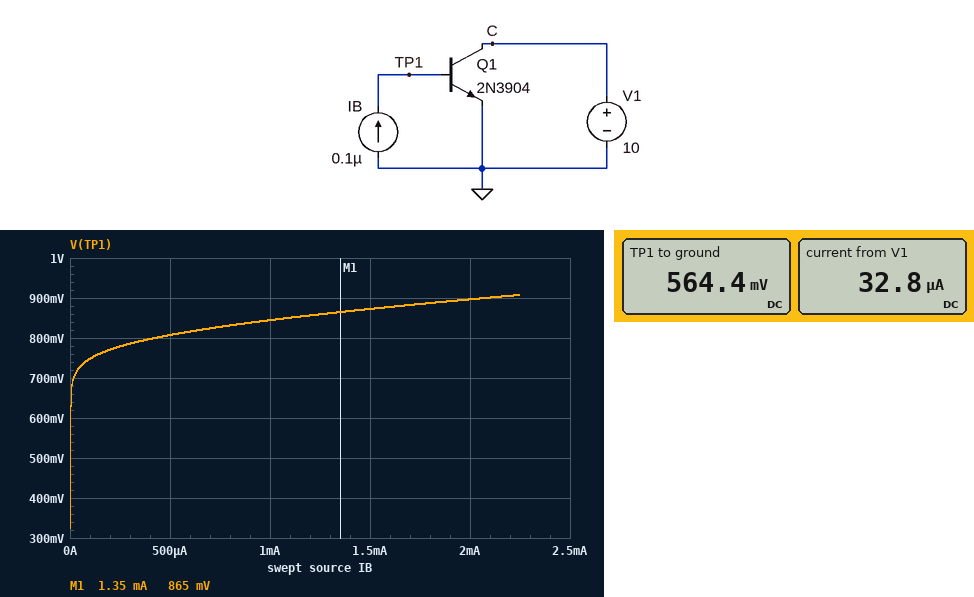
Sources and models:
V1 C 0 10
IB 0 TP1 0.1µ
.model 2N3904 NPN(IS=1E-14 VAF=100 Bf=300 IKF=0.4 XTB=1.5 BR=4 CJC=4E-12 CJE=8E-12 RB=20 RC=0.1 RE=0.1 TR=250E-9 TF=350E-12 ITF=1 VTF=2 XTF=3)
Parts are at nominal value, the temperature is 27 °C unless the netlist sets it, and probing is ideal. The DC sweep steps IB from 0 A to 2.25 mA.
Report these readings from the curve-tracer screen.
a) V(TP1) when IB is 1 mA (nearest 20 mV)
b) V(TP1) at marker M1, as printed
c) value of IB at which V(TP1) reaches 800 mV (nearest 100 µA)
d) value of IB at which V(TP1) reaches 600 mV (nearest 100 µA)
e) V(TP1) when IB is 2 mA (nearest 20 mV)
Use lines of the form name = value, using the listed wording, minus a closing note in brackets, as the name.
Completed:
V(TP1) when IB is 1 mA = 840 mV
V(TP1) at marker M1, as printed = 865 mV
value of IB at which V(TP1) reaches 800 mV = 400 µA
value of IB at which V(TP1) reaches 600 mV = 0 A
V(TP1) when IB is 2 mA = 900 mV
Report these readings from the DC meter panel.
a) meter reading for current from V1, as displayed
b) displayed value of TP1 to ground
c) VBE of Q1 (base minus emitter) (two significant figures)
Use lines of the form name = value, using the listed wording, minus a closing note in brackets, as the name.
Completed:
meter reading for current from V1, as displayed = 32.8 µA
displayed value of TP1 to ground = 564.4 mV
VBE of Q1 (base minus emitter) = 560 mV
